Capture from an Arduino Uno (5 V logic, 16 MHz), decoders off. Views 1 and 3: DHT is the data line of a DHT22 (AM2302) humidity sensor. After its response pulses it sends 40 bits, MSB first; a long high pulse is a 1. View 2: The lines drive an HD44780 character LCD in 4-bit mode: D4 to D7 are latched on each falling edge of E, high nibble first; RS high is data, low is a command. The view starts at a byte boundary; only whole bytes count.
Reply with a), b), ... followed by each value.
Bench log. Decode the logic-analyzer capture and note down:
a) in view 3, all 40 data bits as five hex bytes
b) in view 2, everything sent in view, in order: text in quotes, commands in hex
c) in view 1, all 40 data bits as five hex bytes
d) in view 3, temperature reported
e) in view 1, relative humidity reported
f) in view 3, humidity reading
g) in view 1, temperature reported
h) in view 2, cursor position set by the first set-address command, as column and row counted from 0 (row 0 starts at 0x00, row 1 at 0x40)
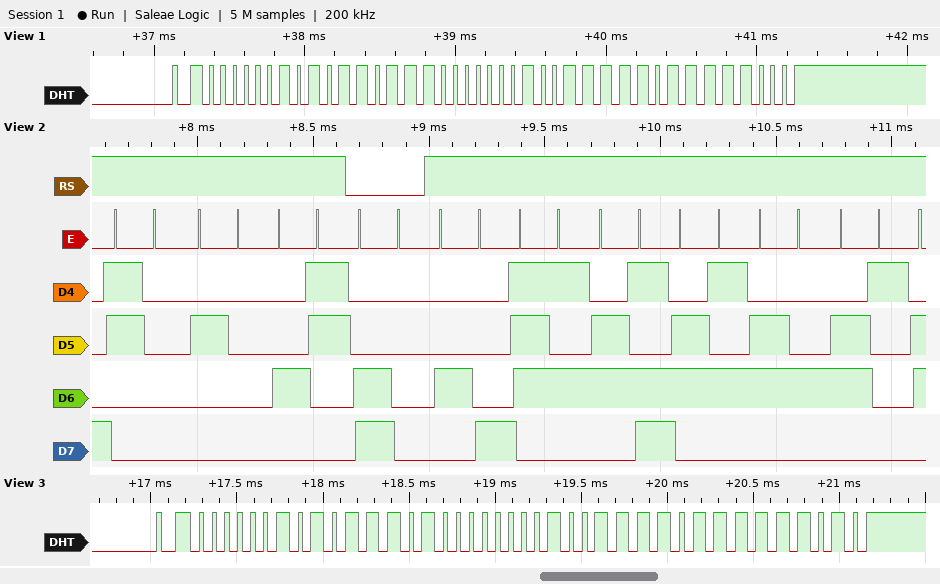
a) 02 BA 01 3D FA
b) "0 C" 0xC0 "Humeda"
c) 02 B7 01 3E F8
d) 31.7 °C
e) 69.5 %
f) 69.8 %
g) 31.8 °C
h) column 0, row 1
